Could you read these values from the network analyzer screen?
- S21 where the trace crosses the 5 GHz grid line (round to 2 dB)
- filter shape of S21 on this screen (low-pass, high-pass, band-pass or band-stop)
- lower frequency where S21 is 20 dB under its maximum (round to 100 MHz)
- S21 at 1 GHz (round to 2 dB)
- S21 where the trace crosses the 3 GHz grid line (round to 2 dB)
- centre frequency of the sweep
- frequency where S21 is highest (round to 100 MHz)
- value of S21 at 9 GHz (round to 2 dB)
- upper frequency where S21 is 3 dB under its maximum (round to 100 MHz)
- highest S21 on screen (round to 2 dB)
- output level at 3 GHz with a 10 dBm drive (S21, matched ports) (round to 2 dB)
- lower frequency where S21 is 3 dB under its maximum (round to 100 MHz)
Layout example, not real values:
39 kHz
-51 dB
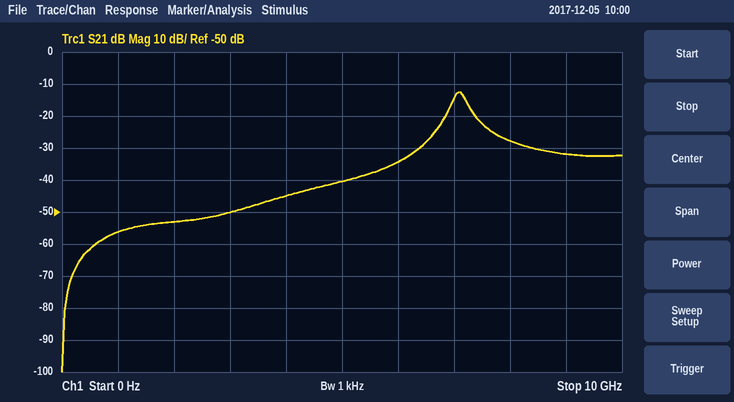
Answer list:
-40 dB
band-pass
6.2 GHz
-56 dB
-50 dB
5 GHz
7.1 GHz
-32 dB
7.2 GHz
-12 dB
-40 dBm
7.0 GHz
